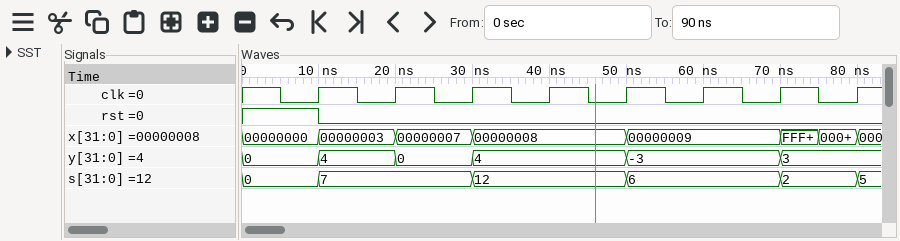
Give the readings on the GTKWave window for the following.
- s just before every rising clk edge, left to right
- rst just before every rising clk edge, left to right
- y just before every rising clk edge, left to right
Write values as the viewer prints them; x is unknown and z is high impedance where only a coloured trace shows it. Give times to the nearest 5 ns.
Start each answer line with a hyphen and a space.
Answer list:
- 0, 7, 7, 12, 12, 6, 6, 2
- 1 0 0 0 0 0 0 0
- 0, 4, 0, 4, 4, -3, -3, 3
